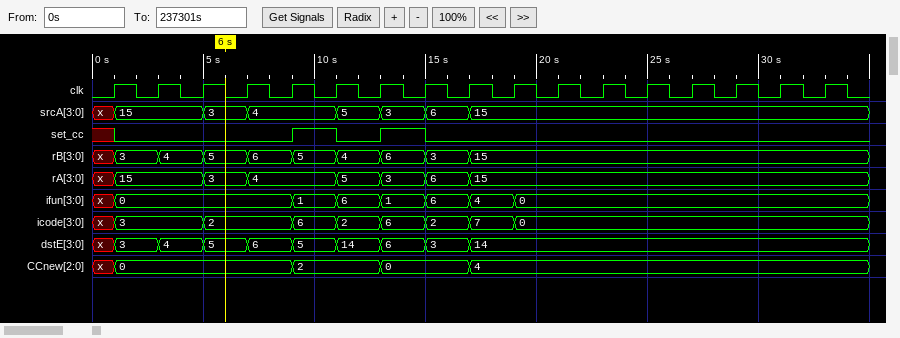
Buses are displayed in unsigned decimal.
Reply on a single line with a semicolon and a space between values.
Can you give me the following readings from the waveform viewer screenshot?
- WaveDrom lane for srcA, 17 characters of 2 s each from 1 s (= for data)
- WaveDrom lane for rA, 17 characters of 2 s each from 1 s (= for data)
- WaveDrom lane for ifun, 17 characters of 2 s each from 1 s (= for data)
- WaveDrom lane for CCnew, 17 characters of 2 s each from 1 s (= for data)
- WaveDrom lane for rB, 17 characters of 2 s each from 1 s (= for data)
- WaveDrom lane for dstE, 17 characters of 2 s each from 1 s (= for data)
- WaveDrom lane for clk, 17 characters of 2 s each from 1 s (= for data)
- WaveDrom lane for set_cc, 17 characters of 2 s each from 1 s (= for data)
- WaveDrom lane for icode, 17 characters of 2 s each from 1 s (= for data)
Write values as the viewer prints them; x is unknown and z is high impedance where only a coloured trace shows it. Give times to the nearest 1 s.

{name: 'srcA', wave: '=.==.====........', data: '15 3 4 5 3 6 15'}; {name: 'rA', wave: '=.==.====........', data: '15 3 4 5 3 6 15'}; {name: 'ifun', wave: '=...======.......', data: '0 1 6 1 6 4 0'}; {name: 'CCnew', wave: '=...=.=.=........', data: '0 2 0 4'}; {name: 'rB', wave: '=========........', data: '3 4 5 6 5 4 6 3 15'}; {name: 'dstE', wave: '=========........', data: '3 4 5 6 5 14 6 3 14'}; {name: 'clk', wave: 'p................'}; {name: 'set_cc', wave: '0...1010.........'}; {name: 'icode', wave: '=.=.======.......', data: '3 2 6 2 6 2 7 0'}
